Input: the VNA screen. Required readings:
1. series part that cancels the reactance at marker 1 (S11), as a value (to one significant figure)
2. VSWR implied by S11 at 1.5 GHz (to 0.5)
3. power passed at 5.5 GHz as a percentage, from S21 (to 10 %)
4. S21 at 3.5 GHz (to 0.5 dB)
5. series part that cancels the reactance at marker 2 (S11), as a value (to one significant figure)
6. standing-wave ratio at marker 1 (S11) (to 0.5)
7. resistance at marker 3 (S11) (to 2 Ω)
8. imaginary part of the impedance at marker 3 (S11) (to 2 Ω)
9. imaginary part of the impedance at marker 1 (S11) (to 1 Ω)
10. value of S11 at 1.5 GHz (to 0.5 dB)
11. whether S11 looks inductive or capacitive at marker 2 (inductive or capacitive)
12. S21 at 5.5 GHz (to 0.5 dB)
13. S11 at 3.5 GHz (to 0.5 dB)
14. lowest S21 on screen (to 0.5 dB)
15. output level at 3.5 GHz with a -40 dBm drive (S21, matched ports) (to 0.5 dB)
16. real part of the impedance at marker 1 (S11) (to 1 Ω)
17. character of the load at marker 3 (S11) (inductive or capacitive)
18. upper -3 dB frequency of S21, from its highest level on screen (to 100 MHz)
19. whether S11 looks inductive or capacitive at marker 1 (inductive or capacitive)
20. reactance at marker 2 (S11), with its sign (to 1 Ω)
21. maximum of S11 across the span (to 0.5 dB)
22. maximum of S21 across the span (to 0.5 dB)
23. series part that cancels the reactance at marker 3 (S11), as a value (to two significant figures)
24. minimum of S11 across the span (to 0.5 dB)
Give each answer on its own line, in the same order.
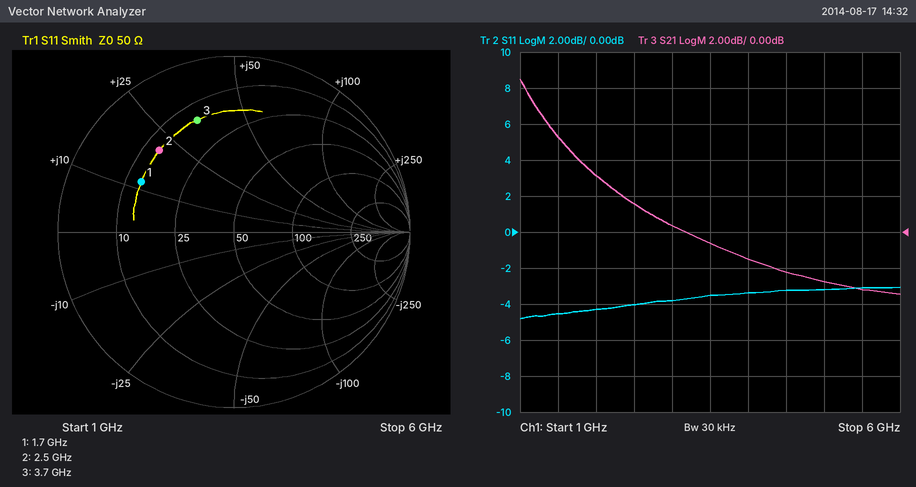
8 pF
4.0
50 %
-0.5 dB
3 pF
4.0
14 Ω
+34 Ω
+12 Ω
-4.5 dB
inductive
-3.0 dB
-3.5 dB
-3.5 dB
-40.5 dBm
13 Ω
inductive
1.5 GHz
inductive
+21 Ω
-3.0 dB
8.5 dB
1.3 pF
-5.0 dB
